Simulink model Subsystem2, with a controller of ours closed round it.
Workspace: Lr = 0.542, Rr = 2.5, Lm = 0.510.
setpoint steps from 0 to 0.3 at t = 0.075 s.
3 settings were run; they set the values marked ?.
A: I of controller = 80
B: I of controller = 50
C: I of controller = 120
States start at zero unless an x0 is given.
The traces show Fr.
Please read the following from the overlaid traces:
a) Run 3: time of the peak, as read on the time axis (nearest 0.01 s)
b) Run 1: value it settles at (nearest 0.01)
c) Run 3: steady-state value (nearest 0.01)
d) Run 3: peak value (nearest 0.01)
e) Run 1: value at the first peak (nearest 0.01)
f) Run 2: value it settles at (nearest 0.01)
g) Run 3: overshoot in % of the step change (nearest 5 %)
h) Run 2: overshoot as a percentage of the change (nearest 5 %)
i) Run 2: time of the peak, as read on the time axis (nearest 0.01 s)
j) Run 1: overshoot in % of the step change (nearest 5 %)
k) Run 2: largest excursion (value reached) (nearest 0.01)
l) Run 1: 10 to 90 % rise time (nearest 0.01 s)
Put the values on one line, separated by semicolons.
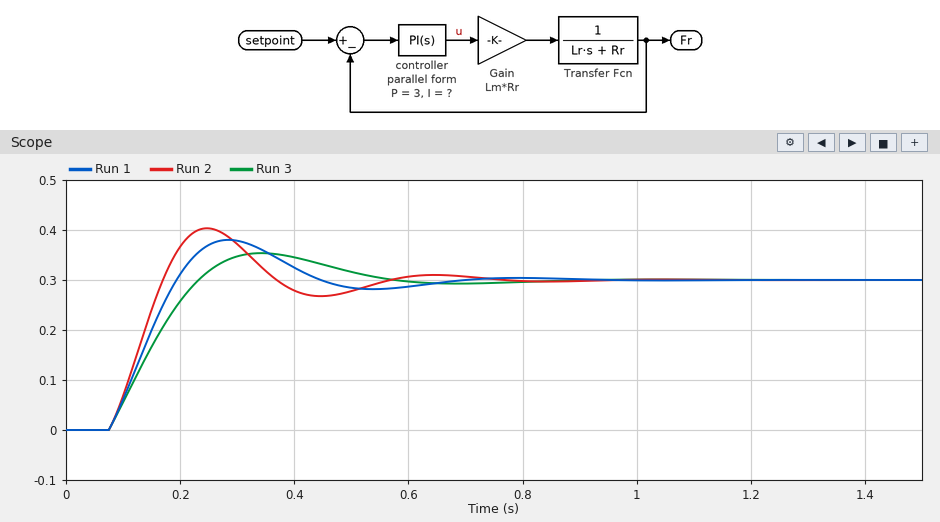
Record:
0.34 s; 0.30; 0.30; 0.35; 0.38; 0.30; 20 %; 35 %; 0.25 s; 25 %; 0.40; 0.09 s
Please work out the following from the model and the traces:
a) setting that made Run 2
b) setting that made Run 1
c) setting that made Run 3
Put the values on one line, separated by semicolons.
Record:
C; A; B
